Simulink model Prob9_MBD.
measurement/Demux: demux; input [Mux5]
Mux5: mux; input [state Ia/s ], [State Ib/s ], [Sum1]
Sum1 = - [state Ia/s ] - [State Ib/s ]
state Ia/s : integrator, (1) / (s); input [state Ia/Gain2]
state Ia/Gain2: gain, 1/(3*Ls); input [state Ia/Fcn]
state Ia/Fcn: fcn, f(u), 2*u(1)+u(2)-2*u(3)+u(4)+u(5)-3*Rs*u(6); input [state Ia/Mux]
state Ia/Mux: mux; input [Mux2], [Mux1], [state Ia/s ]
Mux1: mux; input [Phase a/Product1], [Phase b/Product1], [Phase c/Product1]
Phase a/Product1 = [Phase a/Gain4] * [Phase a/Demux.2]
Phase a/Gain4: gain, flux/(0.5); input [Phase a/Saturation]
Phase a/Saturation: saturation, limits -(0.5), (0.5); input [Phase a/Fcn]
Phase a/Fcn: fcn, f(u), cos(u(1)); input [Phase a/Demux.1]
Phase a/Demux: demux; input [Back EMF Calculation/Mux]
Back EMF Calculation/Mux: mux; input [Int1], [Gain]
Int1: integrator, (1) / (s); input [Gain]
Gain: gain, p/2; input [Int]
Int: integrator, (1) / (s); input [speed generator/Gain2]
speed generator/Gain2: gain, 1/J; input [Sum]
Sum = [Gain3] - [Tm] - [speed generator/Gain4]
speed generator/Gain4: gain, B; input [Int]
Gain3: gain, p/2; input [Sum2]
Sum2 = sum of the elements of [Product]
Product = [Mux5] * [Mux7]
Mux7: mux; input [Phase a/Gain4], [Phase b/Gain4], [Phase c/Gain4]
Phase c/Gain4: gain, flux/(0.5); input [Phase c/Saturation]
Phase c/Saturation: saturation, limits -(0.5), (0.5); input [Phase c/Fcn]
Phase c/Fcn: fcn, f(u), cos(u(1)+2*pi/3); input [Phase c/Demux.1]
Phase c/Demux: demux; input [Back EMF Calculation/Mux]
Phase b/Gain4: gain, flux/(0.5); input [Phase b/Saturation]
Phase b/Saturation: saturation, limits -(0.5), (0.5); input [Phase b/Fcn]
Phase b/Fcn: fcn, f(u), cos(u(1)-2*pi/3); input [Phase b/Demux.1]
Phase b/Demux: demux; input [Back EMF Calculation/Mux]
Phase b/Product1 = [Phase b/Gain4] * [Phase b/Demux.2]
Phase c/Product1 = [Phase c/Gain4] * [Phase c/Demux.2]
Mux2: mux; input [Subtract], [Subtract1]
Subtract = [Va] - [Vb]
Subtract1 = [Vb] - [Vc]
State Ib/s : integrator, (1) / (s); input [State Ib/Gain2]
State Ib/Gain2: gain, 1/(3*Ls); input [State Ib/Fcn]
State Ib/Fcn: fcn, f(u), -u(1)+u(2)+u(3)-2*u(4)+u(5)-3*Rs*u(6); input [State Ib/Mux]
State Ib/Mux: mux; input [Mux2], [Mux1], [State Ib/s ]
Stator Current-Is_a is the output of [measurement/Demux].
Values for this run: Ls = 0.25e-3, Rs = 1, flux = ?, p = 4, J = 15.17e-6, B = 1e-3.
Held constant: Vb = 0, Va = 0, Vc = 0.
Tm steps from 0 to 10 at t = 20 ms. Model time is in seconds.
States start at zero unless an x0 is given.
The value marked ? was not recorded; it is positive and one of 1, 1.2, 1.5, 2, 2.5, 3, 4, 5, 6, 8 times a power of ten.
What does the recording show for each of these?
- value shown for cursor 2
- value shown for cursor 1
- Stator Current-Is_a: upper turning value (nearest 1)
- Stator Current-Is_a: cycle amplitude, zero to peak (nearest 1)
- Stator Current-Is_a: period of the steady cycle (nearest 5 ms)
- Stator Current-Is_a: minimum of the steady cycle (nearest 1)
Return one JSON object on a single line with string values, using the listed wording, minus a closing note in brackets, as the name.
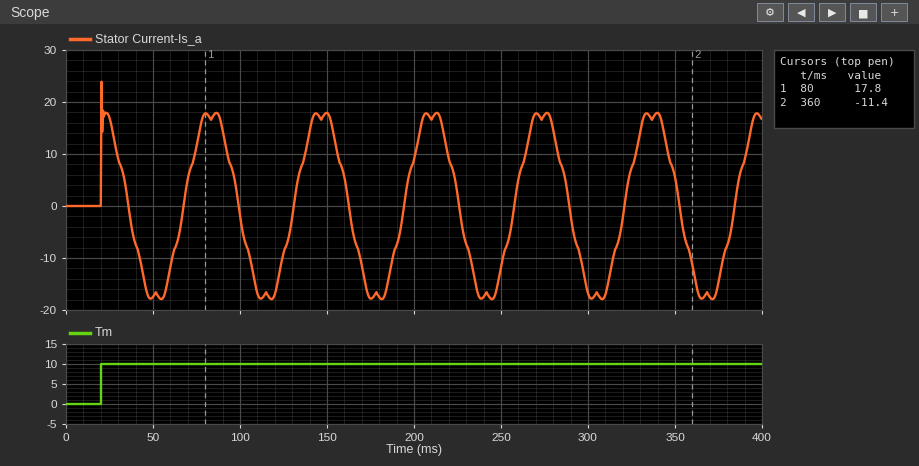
{"value shown for cursor 2": "-11.4", "value shown for cursor 1": "17.8", "Stator Current-Is_a: upper turning value": "18", "Stator Current-Is_a: cycle amplitude, zero to peak": "18", "Stator Current-Is_a: period of the steady cycle": "65 ms", "Stator Current-Is_a: minimum of the steady cycle": "-18"}
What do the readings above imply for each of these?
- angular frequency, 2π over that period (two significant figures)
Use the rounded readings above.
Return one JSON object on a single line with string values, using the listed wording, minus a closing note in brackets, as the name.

{"angular frequency, 2π over that period": "0.097 rad/ms"}
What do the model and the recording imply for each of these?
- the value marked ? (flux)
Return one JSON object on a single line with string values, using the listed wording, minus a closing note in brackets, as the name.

{"the value marked ?": "0.15"}
